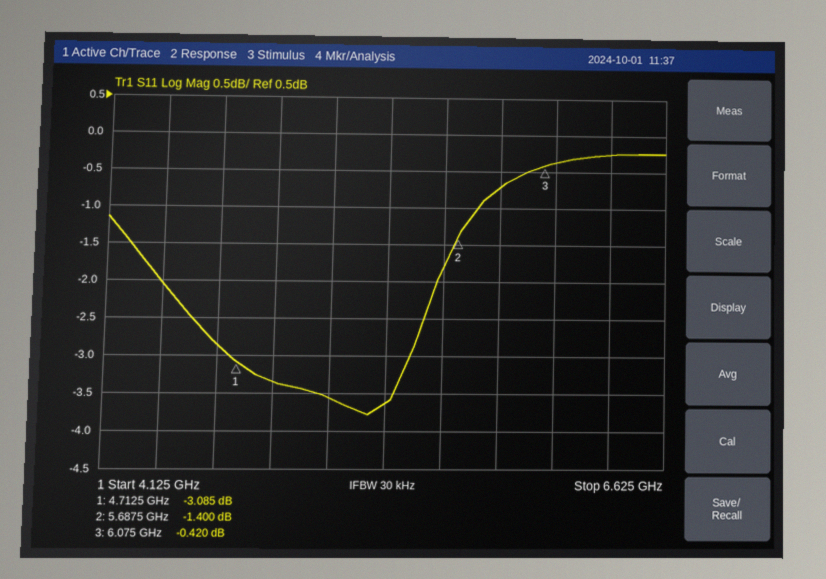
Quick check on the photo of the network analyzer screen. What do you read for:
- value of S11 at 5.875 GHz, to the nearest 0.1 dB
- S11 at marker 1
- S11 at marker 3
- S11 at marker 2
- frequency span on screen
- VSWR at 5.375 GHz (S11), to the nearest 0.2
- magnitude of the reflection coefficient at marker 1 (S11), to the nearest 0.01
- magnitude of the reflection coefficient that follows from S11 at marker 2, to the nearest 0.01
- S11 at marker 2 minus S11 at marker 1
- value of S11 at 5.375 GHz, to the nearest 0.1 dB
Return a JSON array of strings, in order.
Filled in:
["-0.7 dB", "-3.085 dB", "-0.420 dB", "-1.400 dB", "2.5 GHz", "4.8", "0.70", "0.85", "1.685 dB", "-3.6 dB"]
